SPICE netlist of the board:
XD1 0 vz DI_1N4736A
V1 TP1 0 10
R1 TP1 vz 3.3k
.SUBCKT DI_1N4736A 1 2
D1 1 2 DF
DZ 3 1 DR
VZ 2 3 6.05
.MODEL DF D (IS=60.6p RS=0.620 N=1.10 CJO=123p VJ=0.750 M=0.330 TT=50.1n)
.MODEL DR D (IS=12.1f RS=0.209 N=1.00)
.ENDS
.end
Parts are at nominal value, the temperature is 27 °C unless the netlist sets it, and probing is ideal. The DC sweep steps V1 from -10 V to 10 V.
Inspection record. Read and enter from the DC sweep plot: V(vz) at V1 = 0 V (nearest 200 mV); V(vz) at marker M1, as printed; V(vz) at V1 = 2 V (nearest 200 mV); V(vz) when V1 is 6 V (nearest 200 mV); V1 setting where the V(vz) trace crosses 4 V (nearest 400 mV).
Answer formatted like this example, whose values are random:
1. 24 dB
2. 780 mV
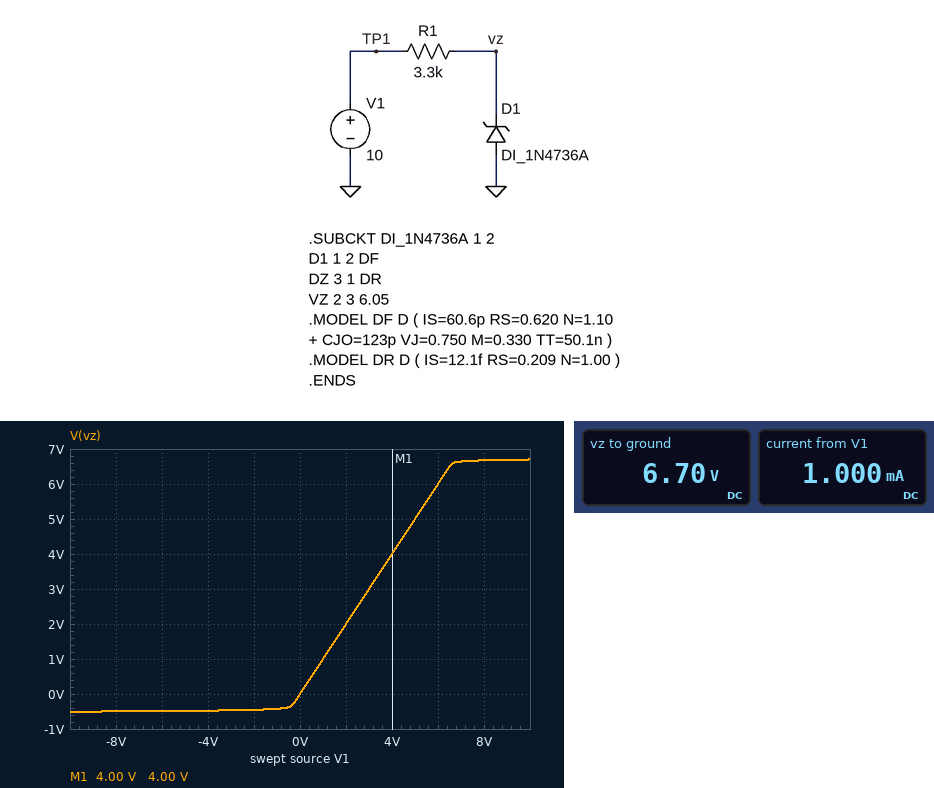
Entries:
1. 0 V
2. 4.00 V
3. 2.0 V
4. 6.0 V
5. 4.0 V
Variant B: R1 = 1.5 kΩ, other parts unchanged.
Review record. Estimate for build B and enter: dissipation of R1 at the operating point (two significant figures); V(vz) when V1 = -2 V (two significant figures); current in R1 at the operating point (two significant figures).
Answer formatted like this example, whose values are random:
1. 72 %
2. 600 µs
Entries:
1. 7.2 mW
2. -470 mV
3. 2.2 mA
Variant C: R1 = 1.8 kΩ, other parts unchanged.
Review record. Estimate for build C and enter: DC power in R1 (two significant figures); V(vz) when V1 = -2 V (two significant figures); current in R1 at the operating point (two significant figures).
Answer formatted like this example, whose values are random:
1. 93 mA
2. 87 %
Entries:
1. 6.0 mW
2. -470 mV
3. 1.8 mA
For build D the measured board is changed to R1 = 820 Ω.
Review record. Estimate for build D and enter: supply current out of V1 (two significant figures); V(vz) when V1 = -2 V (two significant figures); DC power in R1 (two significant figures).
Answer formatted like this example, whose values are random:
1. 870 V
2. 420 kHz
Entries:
1. 4.0 mA
2. -490 mV
3. 13 mW
